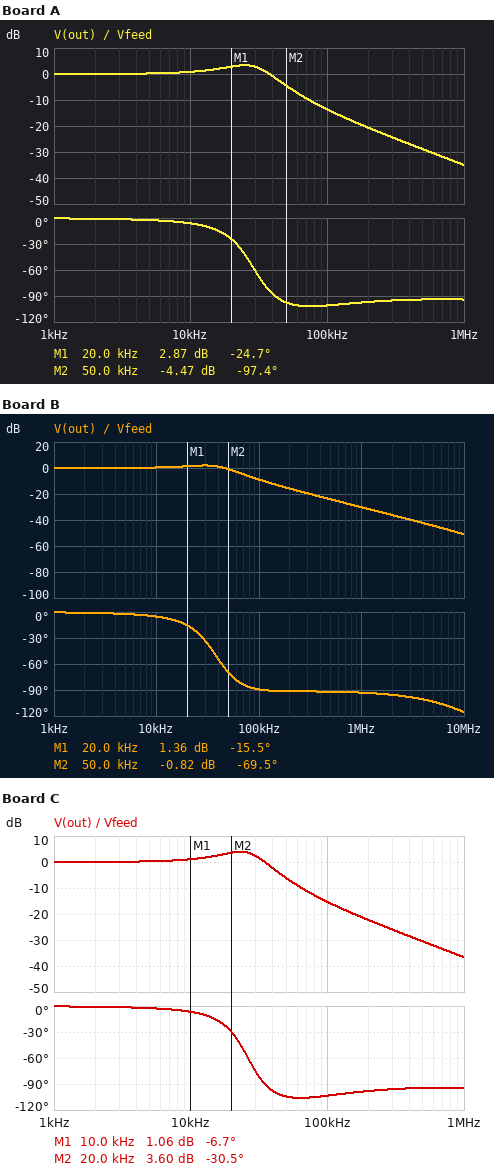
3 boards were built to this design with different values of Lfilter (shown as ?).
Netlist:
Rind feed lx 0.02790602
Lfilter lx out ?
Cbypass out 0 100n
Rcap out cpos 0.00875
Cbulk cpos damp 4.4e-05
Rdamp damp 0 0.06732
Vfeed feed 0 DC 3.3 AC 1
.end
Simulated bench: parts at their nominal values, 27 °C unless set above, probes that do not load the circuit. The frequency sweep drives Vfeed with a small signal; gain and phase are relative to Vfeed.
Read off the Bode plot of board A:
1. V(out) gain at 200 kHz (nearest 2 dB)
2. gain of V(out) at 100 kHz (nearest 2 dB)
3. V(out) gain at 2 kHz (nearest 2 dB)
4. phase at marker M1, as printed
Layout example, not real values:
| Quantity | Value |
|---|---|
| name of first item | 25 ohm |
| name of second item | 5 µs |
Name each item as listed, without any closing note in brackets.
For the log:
| Quantity | Value |
|---|---|
| V(out) gain at 200 kHz | -20 dB |
| gain of V(out) at 100 kHz | -14 dB |
| V(out) gain at 2 kHz | 0 dB |
| phase at marker M1, as printed | -24.7 deg |
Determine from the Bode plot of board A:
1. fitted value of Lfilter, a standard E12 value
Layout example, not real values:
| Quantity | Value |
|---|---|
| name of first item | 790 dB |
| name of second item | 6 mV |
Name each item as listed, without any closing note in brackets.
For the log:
| Quantity | Value |
|---|---|
| fitted value of Lfilter, a standard E12 value | 680 nH |
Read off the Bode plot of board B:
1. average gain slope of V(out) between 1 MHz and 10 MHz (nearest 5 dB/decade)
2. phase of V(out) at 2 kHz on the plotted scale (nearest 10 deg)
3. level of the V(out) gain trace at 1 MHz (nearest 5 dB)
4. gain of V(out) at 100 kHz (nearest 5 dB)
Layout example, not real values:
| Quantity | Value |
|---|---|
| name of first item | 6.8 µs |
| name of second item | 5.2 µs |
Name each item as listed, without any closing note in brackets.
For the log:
| Quantity | Value |
|---|---|
| average gain slope of V(out) between 1 MHz and 10 MHz | -20 dB/decade |
| phase of V(out) at 2 kHz on the plotted scale | 0 deg |
| level of the V(out) gain trace at 1 MHz | -30 dB |
| gain of V(out) at 100 kHz | -10 dB |
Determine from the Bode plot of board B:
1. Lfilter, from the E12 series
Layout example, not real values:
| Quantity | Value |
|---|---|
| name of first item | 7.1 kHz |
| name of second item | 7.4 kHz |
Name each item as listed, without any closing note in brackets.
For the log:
| Quantity | Value |
|---|---|
| Lfilter, from the E12 series | 390 nH |
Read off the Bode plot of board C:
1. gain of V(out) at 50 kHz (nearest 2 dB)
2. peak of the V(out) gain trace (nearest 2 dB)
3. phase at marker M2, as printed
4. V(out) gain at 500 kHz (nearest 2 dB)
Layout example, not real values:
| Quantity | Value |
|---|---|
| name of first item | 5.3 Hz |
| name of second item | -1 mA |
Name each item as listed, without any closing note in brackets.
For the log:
| Quantity | Value |
|---|---|
| gain of V(out) at 50 kHz | -6 dB |
| peak of the V(out) gain trace | 4 dB |
| phase at marker M2, as printed | -30.5 deg |
| V(out) gain at 500 kHz | -30 dB |
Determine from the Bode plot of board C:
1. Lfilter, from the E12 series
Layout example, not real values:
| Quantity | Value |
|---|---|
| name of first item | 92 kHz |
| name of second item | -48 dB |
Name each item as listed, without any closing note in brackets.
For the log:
| Quantity | Value |
|---|---|
| Lfilter, from the E12 series | 820 nH |
